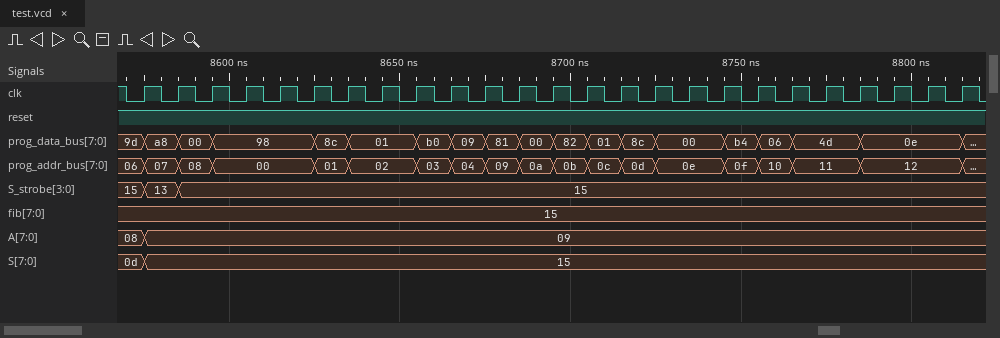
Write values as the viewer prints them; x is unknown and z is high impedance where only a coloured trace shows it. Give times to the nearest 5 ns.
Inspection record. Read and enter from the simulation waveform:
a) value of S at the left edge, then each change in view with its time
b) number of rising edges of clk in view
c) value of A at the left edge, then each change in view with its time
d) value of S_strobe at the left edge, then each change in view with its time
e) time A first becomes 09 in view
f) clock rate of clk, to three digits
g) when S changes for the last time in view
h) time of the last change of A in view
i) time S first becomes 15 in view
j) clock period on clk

0d, 15 at 8575 ns
25
08, 09 at 8575 ns
15, 13 at 8575 ns, 15 at 8585 ns
8575 ns
100 MHz
8575 ns
8575 ns
8575 ns
10 ns
